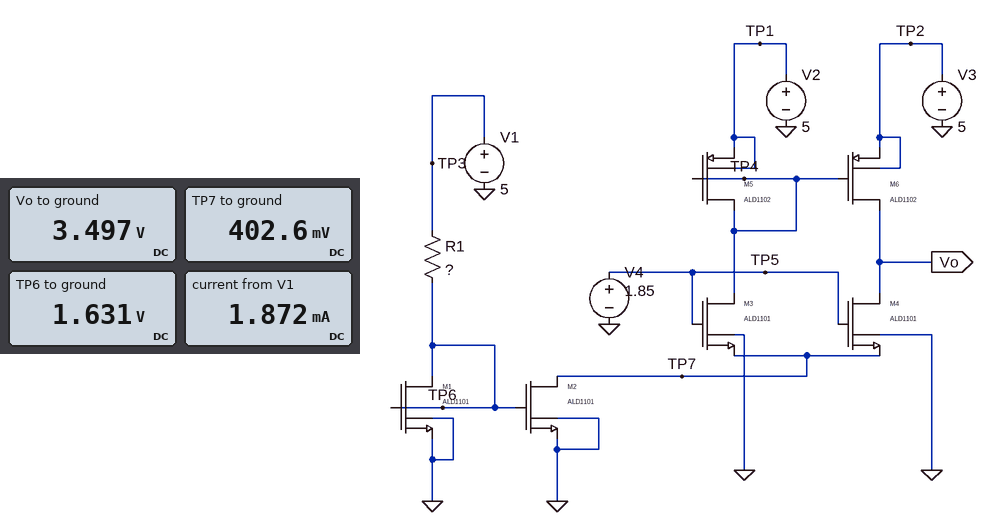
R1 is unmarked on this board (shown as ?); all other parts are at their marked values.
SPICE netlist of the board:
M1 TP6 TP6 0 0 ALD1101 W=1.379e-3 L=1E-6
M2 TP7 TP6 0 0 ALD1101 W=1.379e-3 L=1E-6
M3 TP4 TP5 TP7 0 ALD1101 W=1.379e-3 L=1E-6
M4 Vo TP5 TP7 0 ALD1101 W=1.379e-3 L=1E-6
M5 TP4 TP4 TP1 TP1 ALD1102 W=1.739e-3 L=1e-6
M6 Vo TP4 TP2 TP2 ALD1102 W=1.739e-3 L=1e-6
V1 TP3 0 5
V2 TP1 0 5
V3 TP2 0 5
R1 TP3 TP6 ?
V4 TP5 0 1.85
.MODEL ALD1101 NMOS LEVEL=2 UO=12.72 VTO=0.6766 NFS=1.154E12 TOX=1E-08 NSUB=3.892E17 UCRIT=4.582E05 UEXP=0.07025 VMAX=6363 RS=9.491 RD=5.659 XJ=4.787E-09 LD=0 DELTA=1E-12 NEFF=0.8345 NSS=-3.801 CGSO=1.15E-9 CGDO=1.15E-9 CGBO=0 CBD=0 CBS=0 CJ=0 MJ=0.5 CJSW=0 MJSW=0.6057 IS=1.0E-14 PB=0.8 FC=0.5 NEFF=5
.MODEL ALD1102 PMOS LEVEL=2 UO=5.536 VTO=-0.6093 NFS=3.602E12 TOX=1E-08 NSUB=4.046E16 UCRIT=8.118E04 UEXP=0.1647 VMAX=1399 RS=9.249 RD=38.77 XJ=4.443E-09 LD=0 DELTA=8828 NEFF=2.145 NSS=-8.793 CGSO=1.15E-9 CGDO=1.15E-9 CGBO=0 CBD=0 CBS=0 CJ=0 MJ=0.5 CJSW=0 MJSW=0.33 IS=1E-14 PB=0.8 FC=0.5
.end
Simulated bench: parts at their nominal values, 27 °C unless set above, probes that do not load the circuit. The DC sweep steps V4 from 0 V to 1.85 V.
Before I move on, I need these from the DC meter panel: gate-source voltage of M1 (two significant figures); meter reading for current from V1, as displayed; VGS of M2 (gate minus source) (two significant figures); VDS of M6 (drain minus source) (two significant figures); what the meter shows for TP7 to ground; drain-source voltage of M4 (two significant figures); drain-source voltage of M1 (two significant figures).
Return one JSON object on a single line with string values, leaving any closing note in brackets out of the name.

{"gate-source voltage of M1": "1.6 V", "meter reading for current from V1, as displayed": "1.872 mA", "VGS of M2 (gate minus source)": "1.6 V", "VDS of M6 (drain minus source)": "-1.5 V", "what the meter shows for TP7 to ground": "402.6 mV", "drain-source voltage of M4": "3.1 V", "drain-source voltage of M1": "1.6 V"}
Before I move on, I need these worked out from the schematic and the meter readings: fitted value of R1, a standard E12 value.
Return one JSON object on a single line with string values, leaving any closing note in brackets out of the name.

{"fitted value of R1, a standard E12 value": "1.8 kΩ"}
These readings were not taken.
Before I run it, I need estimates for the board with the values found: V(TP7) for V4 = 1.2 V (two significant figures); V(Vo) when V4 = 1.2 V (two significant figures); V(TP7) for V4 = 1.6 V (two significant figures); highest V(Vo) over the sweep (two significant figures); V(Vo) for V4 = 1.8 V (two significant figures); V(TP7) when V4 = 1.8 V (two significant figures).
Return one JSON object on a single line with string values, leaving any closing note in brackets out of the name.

{"V(TP7) for V4 = 1.2 V": "120 mV", "V(Vo) when V4 = 1.2 V": "3.8 V", "V(TP7) for V4 = 1.6 V": "280 mV", "highest V(Vo) over the sweep": "5.0 V", "V(Vo) for V4 = 1.8 V": "3.5 V", "V(TP7) when V4 = 1.8 V": "380 mV"}
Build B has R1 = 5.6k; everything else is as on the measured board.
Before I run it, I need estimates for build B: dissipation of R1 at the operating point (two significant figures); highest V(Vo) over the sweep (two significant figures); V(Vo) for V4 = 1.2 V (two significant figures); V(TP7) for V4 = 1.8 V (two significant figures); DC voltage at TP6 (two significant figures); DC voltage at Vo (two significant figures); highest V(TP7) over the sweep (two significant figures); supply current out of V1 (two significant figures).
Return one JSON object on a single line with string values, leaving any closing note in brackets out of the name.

{"dissipation of R1 at the operating point": "2.5 mW", "highest V(Vo) over the sweep": "5.0 V", "V(Vo) for V4 = 1.2 V": "3.9 V", "V(TP7) for V4 = 1.8 V": "510 mV", "DC voltage at TP6": "1.2 V", "DC voltage at Vo": "3.8 V", "highest V(TP7) over the sweep": "550 mV", "supply current out of V1": "670 µA"}
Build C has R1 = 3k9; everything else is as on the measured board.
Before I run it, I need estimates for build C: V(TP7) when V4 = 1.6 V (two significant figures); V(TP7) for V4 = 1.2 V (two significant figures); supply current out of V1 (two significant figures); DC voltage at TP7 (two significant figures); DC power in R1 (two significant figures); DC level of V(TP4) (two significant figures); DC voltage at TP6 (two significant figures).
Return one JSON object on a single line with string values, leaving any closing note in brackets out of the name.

{"V(TP7) when V4 = 1.6 V": "340 mV", "V(TP7) for V4 = 1.2 V": "140 mV", "supply current out of V1": "940 µA", "DC voltage at TP7": "500 mV", "DC power in R1": "3.4 mW", "DC level of V(TP4)": "3.7 V", "DC voltage at TP6": "1.3 V"}
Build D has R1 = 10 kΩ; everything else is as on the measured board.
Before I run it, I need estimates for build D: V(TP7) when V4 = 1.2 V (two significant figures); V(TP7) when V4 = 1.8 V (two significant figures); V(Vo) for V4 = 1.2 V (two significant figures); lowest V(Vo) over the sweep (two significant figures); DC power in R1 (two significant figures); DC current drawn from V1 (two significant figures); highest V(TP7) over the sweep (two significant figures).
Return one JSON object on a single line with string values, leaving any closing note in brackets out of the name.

{"V(TP7) when V4 = 1.2 V": "180 mV", "V(TP7) when V4 = 1.8 V": "580 mV", "V(Vo) for V4 = 1.2 V": "4.0 V", "lowest V(Vo) over the sweep": "3.9 V", "DC power in R1": "1.5 mW", "DC current drawn from V1": "390 µA", "highest V(TP7) over the sweep": "620 mV"}
